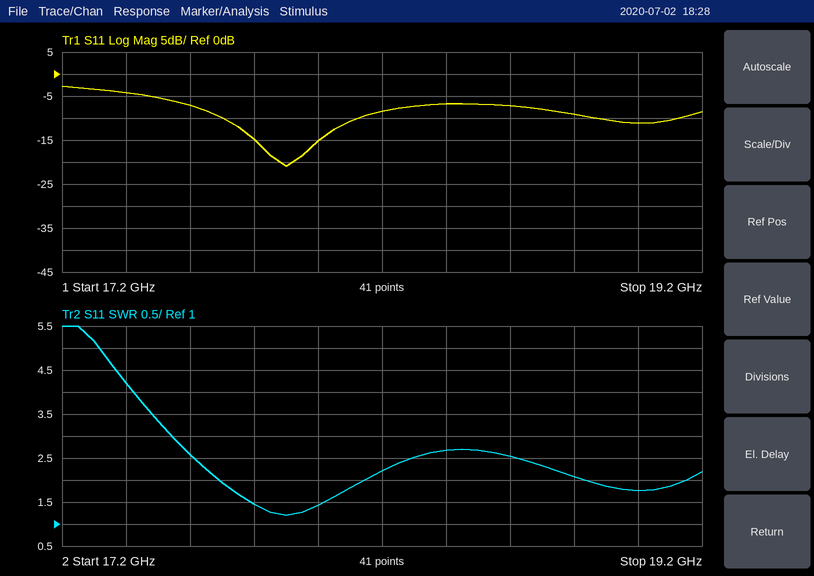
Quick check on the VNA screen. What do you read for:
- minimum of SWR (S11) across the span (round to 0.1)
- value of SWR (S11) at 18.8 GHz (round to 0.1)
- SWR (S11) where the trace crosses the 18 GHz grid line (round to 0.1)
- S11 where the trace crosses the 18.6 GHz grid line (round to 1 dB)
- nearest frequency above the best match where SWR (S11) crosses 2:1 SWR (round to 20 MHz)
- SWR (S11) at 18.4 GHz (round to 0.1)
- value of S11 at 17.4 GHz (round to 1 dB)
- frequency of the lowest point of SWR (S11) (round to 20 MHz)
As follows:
1.2
2.1
1.4
-7 dB
18.14 GHz
2.7
-4 dB
17.90 GHz
